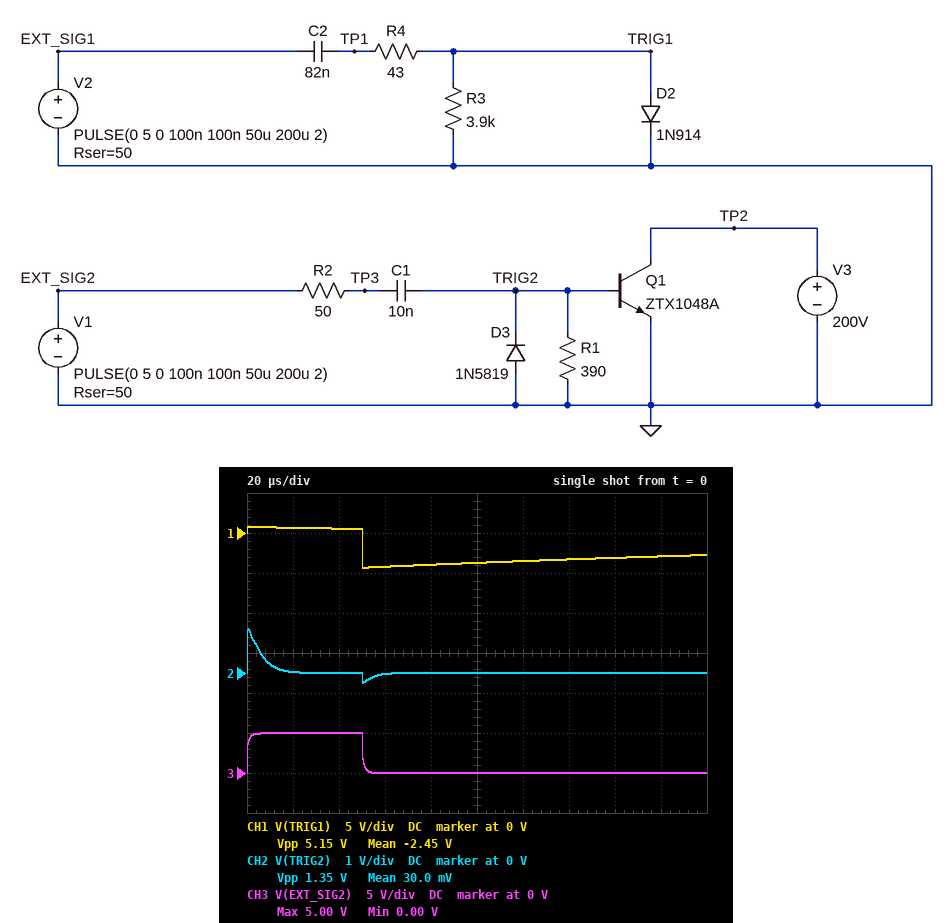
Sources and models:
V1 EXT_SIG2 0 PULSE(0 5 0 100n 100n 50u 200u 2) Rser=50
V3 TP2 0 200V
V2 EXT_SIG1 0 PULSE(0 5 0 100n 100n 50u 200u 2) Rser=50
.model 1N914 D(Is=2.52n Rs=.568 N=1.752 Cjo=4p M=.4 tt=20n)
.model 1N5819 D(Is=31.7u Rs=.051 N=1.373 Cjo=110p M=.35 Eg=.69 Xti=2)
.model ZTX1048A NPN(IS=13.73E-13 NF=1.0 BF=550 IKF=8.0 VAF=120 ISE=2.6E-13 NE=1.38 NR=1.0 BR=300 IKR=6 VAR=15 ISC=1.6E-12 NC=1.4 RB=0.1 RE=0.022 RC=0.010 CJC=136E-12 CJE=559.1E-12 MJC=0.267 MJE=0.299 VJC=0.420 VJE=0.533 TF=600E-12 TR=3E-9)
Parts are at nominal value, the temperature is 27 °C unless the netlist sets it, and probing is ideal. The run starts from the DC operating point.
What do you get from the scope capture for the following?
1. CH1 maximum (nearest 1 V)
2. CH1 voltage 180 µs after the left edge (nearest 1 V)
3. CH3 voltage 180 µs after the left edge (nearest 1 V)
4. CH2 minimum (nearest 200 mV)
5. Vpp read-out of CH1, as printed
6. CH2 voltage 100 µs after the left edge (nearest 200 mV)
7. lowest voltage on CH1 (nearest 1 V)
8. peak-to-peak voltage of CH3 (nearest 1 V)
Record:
1 V
-3 V
0 V
-200 mV
5.15 V
0 V
-4 V
5 V
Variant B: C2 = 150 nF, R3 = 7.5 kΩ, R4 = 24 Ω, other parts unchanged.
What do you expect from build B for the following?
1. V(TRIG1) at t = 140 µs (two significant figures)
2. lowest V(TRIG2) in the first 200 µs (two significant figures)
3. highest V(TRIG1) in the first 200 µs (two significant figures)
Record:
-4.0 V
-260 mV
800 mV
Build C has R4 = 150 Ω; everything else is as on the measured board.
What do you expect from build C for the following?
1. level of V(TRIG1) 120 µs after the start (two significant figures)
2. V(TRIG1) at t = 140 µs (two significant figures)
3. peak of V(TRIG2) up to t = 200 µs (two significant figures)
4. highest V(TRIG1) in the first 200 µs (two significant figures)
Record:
-3.2 V
-3.0 V
1.1 V
730 mV
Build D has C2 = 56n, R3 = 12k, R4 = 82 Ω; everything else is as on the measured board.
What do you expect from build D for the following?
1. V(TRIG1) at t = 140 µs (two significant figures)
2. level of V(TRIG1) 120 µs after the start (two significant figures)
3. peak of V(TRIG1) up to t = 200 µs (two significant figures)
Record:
-3.9 V
-4.0 V
760 mV
